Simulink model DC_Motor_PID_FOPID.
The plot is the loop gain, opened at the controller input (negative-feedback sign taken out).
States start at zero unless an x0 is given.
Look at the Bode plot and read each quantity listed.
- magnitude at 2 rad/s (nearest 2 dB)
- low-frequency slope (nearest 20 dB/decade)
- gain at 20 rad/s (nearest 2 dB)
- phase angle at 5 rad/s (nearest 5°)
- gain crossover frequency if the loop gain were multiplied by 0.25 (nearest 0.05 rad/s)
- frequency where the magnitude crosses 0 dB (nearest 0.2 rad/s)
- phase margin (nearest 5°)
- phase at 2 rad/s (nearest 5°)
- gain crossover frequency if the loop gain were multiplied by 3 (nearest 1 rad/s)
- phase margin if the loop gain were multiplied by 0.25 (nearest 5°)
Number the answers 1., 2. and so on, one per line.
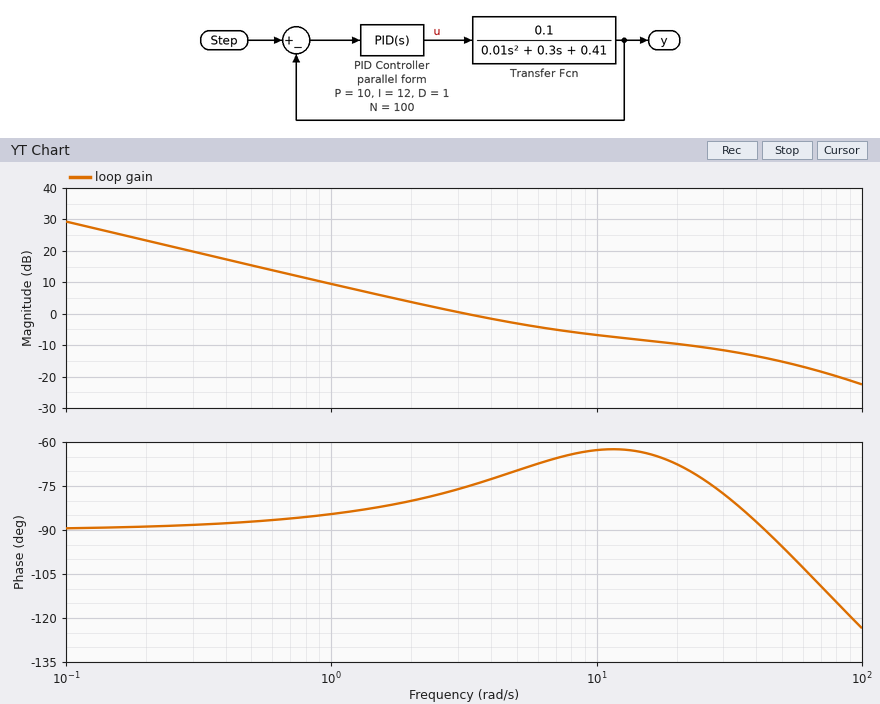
1. 4 dB
2. -20 dB/decade
3. -10 dB
4. -70°
5. 0.75 rad/s
6. 3.2 rad/s
7. 105°
8. -80°
9. 20 rad/s
10. 95°
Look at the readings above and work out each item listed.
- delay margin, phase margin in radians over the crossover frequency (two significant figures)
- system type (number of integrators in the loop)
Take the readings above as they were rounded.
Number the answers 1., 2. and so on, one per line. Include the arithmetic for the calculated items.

1. 105 × π / 180 / 3.2 = 0.57 s
2. 1
